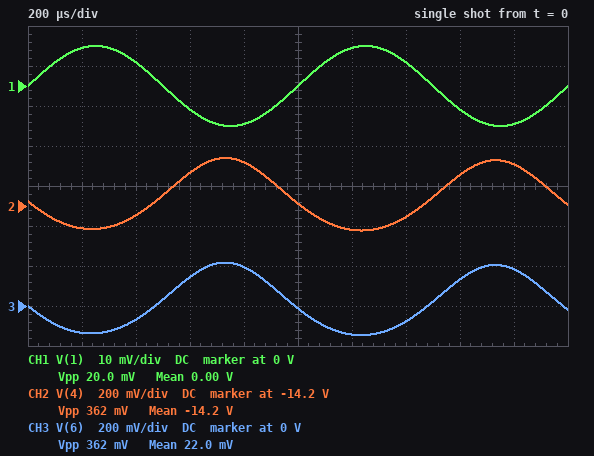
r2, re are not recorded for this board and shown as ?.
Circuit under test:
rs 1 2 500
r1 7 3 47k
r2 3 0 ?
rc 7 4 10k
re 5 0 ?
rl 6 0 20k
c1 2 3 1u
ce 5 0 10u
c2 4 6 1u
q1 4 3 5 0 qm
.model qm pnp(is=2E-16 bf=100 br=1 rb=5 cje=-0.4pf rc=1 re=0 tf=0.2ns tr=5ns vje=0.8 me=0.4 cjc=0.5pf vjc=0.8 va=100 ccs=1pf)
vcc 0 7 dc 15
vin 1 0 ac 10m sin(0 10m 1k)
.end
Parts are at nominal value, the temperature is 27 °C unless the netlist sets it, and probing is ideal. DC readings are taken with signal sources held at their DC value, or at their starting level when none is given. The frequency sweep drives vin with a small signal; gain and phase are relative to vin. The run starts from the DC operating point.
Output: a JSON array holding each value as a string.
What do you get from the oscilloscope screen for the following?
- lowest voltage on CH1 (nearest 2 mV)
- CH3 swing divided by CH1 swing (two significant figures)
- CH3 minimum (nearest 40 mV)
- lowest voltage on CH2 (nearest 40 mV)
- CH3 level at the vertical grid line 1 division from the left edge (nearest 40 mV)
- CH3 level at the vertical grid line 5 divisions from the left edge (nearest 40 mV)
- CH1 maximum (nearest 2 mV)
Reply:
["-10 mV", "18", "-160 mV", "-14.32 V", "-120 mV", "0 V", "10 mV"]
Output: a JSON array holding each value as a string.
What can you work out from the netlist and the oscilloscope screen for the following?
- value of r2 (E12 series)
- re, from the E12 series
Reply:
["2.7 kΩ", "1.5 kΩ"]
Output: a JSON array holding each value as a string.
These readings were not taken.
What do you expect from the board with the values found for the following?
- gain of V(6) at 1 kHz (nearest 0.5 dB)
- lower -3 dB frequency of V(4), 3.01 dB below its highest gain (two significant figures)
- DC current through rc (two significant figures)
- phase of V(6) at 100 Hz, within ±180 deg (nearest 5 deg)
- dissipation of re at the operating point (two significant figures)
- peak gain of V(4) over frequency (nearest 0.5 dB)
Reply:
["25.0 dB", "90 Hz", "82 µA", "-125 deg", "10 µW", "25.0 dB"]
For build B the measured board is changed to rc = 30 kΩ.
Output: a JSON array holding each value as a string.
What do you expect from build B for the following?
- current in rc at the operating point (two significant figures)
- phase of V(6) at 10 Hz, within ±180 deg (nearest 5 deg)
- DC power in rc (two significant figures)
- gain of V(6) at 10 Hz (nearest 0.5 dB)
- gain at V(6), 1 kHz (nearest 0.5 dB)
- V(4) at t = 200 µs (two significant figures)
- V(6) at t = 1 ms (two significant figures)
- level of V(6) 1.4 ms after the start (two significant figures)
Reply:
["82 µA", "-50 deg", "200 µW", "2.5 dB", "30.0 dB", "-13 V", "-21 mV", "-140 mV"]
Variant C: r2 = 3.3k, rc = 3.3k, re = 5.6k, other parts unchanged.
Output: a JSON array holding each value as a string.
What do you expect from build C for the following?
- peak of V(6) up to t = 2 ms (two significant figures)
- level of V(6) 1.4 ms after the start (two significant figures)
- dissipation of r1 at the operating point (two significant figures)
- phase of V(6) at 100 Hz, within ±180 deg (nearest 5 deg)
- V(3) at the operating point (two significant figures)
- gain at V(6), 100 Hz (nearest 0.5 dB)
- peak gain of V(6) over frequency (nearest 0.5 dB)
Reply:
["63 mV", "-23 mV", "4.2 mW", "-135 deg", "-980 mV", "12.5 dB", "14.0 dB"]
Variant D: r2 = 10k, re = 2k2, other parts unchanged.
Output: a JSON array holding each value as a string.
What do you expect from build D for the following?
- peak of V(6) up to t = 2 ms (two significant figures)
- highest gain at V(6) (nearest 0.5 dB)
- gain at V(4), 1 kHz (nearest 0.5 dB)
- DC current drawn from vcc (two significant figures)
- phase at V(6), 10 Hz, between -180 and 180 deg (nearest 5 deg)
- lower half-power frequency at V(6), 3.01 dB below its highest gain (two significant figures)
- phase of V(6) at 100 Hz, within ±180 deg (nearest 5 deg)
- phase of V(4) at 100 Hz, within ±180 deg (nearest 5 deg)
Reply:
["1.7 V", "44.5 dB", "43.5 dB", "1.1 mA", "-40 deg", "470 Hz", "-95 deg", "-100 deg"]
